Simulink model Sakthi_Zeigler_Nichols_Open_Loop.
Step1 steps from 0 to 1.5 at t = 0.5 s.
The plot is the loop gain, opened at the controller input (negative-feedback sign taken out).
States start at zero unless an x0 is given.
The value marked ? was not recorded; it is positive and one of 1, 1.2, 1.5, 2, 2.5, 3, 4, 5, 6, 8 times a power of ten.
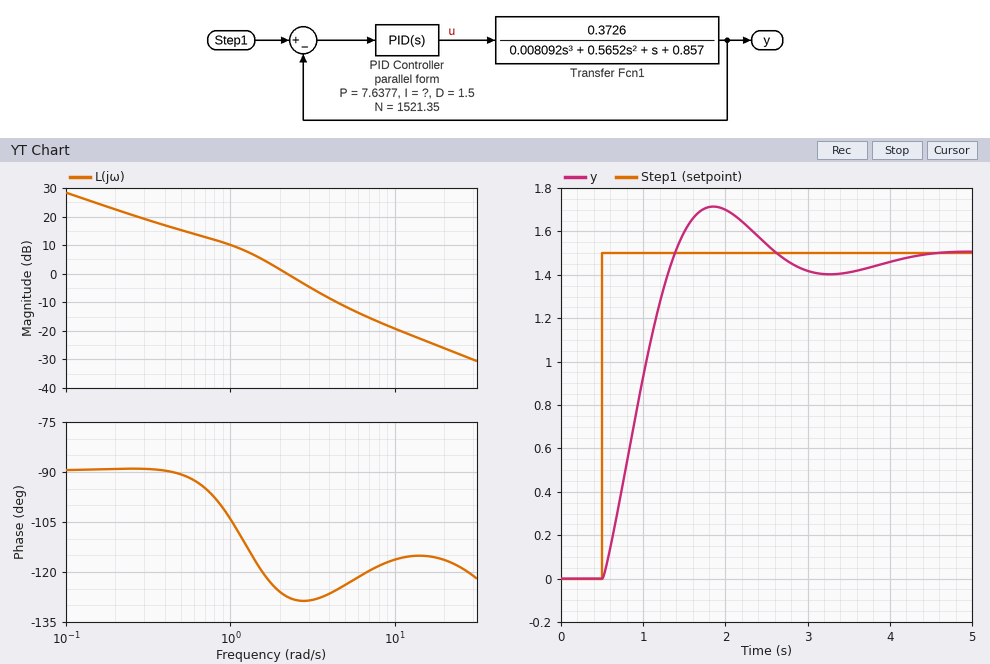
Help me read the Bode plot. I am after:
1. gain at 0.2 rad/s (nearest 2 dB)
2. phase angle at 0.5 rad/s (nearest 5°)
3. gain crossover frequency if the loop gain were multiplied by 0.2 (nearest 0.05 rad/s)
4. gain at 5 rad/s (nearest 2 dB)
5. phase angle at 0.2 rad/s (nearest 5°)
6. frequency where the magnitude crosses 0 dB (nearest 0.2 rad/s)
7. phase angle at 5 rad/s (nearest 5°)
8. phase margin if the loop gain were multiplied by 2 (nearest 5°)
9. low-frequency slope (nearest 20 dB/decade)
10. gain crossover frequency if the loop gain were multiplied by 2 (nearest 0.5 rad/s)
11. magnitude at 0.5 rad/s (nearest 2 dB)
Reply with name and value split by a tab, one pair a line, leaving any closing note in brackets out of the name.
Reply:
gain at 0.2 rad/s	22 dB
phase angle at 0.5 rad/s	-90°
gain crossover frequency if the loop gain were multiplied by 0.2	0.60 rad/s
gain at 5 rad/s	-12 dB
phase angle at 0.2 rad/s	-90°
frequency where the magnitude crosses 0 dB	2.2 rad/s
phase angle at 5 rad/s	-125°
phase margin if the loop gain were multiplied by 2	50°
low-frequency slope	-20 dB/decade
gain crossover frequency if the loop gain were multiplied by 2	3.5 rad/s
magnitude at 0.5 rad/s	16 dB
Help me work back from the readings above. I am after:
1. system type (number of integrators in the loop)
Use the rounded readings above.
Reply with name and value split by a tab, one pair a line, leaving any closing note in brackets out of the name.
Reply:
system type	1
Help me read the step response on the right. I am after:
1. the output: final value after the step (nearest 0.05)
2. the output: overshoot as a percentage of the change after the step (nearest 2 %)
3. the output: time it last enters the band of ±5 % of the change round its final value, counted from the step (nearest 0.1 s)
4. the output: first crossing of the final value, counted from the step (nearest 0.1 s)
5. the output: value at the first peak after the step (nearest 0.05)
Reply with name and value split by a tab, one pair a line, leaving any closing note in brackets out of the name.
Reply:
the output: final value after the step	1.50
the output: overshoot as a percentage of the change after the step	14 %
the output: time it last enters the band of ±5 % of the change round its final value, counted from the step	3.2 s
the output: first crossing of the final value, counted from the step	0.9 s
the output: value at the first peak after the step	1.70
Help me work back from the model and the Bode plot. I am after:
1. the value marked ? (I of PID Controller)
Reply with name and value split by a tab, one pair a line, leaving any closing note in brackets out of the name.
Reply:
the value marked ?	6
